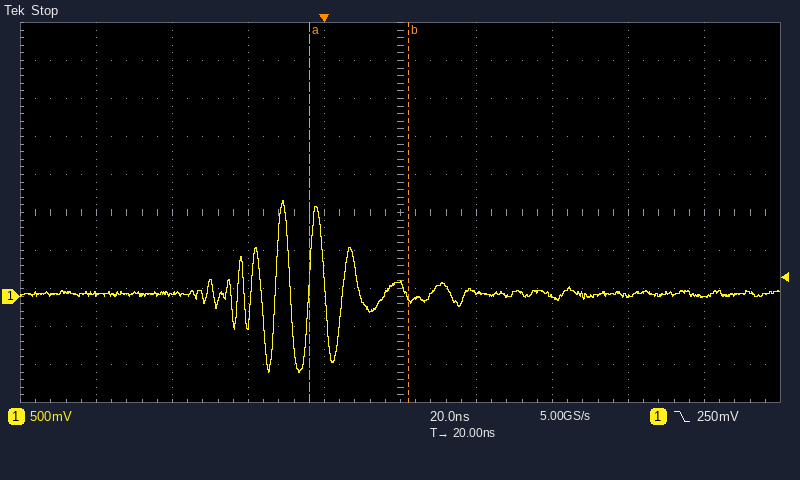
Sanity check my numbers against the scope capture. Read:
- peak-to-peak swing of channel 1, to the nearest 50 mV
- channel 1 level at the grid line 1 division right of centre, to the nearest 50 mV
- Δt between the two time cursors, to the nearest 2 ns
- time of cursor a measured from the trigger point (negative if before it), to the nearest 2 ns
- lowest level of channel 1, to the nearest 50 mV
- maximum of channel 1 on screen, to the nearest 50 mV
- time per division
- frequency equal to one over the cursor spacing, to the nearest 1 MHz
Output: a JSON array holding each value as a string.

["2.25 V", "50 mV", "26 ns", "-4 ns", "-1.00 V", "1.25 V", "20 ns", "38 MHz"]
